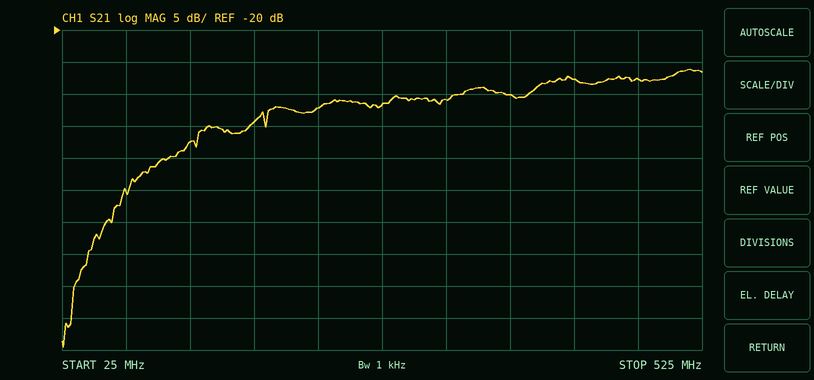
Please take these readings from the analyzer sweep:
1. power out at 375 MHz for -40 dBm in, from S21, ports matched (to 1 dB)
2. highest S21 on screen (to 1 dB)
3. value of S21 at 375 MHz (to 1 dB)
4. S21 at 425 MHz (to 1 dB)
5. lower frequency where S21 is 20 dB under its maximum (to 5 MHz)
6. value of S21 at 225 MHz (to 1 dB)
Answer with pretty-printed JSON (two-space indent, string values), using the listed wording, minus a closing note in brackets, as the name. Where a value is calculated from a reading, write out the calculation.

{
  "power out at 375 MHz for -40 dBm in, from S21, ports matched": "-40 dBm + (-30 dB) = -70 dBm",
  "highest S21 on screen": "-26 dB",
  "value of S21 at 375 MHz": "-30 dB",
  "S21 at 425 MHz": "-28 dB",
  "lower frequency where S21 is 20 dB under its maximum": "70 MHz",
  "value of S21 at 225 MHz": "-32 dB"
}
